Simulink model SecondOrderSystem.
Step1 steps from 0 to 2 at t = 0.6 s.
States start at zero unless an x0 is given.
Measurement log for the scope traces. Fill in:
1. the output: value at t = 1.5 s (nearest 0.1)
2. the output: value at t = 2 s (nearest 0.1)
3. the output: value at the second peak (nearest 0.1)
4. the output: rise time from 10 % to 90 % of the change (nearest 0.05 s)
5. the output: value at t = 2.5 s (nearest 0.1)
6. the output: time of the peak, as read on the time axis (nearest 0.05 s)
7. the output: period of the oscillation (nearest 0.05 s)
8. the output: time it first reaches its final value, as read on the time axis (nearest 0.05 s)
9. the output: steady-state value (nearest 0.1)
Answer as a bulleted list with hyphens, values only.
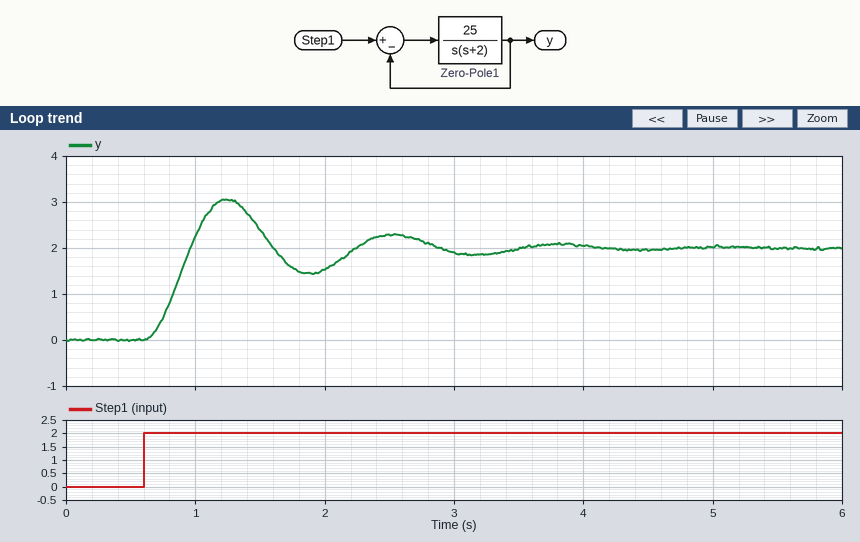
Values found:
- 2.4
- 1.5
- 2.3
- 0.25 s
- 2.3
- 1.25 s
- 1.30 s
- 0.95 s
- 2.0
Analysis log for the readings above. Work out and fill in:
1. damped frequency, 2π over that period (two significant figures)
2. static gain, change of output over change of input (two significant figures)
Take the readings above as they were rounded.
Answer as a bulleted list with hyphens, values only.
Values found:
- 4.8 rad/s
- 1.0
